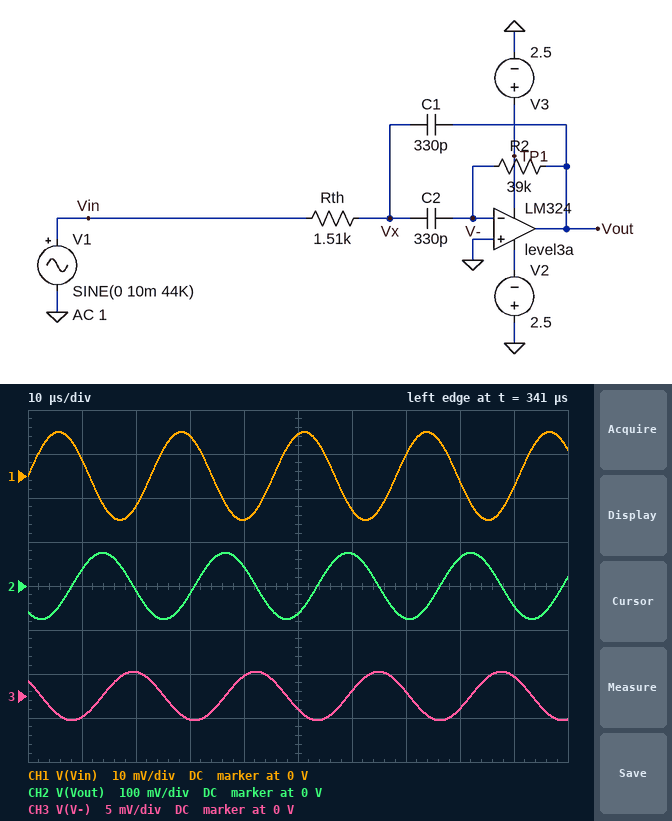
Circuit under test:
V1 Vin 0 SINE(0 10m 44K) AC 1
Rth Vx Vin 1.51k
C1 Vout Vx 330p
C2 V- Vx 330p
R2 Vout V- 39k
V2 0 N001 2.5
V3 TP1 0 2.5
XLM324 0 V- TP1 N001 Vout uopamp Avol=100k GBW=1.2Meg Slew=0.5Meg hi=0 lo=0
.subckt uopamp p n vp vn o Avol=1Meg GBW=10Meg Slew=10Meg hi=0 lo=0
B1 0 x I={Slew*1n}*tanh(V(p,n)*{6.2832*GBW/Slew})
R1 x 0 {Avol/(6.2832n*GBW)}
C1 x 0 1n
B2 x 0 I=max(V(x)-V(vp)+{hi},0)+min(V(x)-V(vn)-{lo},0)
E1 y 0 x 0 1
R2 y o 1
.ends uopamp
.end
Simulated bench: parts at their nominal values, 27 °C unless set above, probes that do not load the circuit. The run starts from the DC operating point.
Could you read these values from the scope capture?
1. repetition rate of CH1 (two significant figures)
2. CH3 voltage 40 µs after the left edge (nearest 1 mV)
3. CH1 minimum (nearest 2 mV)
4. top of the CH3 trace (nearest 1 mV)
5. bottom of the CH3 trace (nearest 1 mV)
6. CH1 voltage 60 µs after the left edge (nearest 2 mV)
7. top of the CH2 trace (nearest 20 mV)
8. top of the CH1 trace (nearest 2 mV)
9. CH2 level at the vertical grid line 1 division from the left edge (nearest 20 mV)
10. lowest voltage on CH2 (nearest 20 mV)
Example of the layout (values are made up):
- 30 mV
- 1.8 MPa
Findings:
- 44 kHz
- 2 mV
- -10 mV
- 3 mV
- -3 mV
- -8 mV
- 80 mV
- 10 mV
- 40 mV
- -80 mV
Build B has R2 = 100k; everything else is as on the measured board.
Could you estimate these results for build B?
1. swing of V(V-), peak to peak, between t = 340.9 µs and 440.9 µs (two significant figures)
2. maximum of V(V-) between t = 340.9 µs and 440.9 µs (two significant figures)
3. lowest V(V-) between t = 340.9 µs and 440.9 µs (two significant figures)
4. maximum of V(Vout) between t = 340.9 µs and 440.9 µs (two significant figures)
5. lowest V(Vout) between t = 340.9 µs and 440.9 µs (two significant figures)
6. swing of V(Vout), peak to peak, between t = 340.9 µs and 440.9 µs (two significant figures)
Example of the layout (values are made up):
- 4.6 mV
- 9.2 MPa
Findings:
- 10 mV
- 5.1 mV
- -5.1 mV
- 140 mV
- -140 mV
- 280 mV
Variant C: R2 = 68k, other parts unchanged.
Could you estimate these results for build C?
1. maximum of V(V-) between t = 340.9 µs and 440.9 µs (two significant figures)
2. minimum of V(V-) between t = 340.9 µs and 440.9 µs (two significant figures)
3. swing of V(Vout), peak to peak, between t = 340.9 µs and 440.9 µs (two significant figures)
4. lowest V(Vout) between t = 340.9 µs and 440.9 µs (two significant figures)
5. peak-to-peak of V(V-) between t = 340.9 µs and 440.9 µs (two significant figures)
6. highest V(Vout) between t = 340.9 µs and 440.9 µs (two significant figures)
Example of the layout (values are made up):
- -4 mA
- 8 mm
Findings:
- 7.7 mV
- -7.7 mV
- 420 mV
- -210 mV
- 15 mV
- 210 mV
